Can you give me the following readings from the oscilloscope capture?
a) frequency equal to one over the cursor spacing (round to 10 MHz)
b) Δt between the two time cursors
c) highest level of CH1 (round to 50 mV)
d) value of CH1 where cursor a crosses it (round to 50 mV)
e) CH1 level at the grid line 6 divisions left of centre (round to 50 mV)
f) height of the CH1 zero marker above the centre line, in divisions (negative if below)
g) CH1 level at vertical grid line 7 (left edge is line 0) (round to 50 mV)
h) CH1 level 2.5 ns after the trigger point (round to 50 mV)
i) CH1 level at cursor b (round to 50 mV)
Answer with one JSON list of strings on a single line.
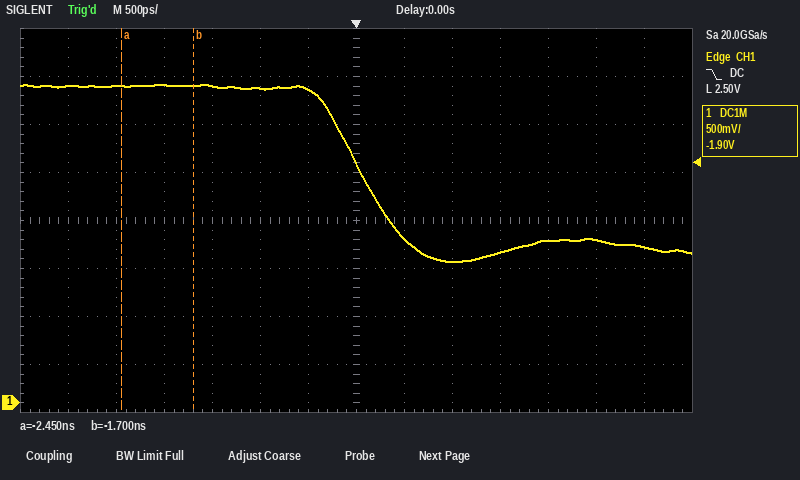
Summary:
["1.33 GHz", "750 ps", "3.30 V", "3.30 V", "3.30 V", "-3.8 div", "2.50 V", "1.70 V", "3.30 V"]
